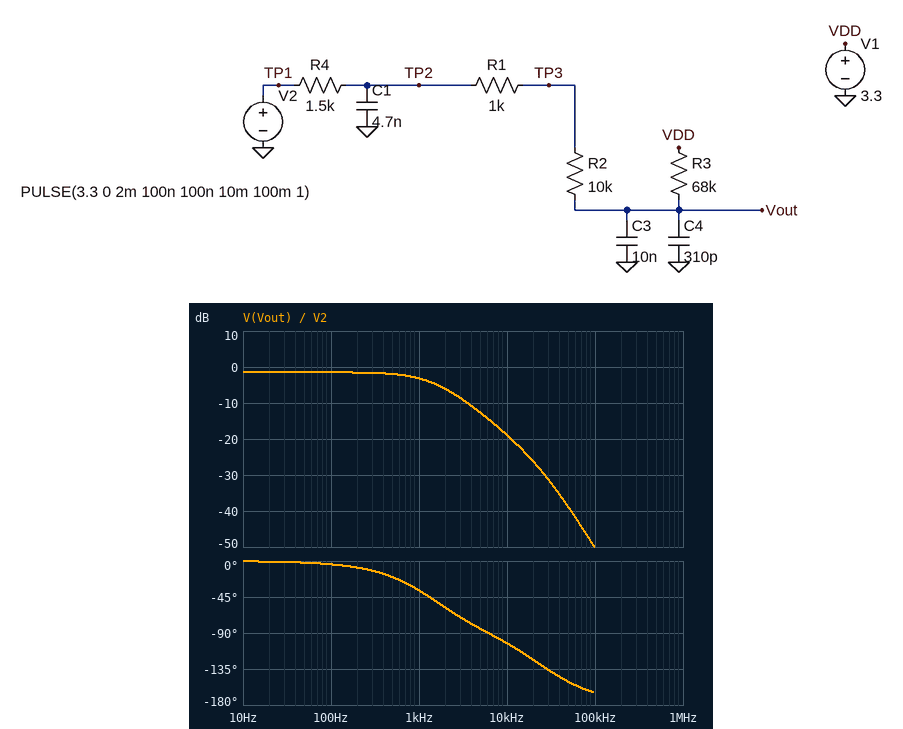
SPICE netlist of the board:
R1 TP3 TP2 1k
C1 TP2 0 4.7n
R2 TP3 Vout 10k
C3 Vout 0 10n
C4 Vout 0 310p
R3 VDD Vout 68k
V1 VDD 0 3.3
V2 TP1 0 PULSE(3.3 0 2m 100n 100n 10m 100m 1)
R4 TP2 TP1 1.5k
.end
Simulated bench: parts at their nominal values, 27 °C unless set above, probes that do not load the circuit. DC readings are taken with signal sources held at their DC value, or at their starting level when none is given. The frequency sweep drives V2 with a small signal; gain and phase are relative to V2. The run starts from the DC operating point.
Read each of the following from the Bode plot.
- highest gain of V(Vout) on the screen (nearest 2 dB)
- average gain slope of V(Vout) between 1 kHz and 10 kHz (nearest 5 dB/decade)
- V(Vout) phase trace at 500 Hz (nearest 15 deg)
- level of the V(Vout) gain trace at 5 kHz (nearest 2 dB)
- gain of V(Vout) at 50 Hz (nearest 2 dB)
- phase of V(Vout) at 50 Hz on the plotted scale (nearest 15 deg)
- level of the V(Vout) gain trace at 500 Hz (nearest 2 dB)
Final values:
-2 dB
-15 dB/decade
-15 deg
-12 dB
-2 dB
0 deg
-2 dB
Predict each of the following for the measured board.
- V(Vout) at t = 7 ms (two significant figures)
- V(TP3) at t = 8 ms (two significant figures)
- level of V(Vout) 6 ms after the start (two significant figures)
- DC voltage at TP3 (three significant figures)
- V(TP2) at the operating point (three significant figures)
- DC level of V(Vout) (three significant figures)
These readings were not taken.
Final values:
510 mV
100 mV
510 mV
3.30 V
3.30 V
3.30 V
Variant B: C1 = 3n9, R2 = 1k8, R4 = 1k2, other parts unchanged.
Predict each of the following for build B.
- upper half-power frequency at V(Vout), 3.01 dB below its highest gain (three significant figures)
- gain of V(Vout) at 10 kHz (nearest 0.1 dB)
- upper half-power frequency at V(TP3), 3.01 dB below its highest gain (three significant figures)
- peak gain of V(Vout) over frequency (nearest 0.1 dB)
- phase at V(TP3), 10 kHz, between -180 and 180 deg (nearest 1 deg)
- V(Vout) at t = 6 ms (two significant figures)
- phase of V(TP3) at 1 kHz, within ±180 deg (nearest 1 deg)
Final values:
3.92 kHz
-9.4 dB
5.02 kHz
-0.5 dB
-31 deg
180 mV
-9 deg
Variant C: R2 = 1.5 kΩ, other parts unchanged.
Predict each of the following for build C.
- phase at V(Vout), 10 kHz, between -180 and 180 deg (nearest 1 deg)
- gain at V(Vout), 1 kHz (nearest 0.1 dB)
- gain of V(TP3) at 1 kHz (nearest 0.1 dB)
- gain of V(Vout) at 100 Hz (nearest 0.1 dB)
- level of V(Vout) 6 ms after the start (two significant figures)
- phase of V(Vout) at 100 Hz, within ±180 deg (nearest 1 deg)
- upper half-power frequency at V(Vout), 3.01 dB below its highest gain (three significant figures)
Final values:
-84 deg
-0.8 dB
-0.6 dB
-0.5 dB
180 mV
-2 deg
3.78 kHz
